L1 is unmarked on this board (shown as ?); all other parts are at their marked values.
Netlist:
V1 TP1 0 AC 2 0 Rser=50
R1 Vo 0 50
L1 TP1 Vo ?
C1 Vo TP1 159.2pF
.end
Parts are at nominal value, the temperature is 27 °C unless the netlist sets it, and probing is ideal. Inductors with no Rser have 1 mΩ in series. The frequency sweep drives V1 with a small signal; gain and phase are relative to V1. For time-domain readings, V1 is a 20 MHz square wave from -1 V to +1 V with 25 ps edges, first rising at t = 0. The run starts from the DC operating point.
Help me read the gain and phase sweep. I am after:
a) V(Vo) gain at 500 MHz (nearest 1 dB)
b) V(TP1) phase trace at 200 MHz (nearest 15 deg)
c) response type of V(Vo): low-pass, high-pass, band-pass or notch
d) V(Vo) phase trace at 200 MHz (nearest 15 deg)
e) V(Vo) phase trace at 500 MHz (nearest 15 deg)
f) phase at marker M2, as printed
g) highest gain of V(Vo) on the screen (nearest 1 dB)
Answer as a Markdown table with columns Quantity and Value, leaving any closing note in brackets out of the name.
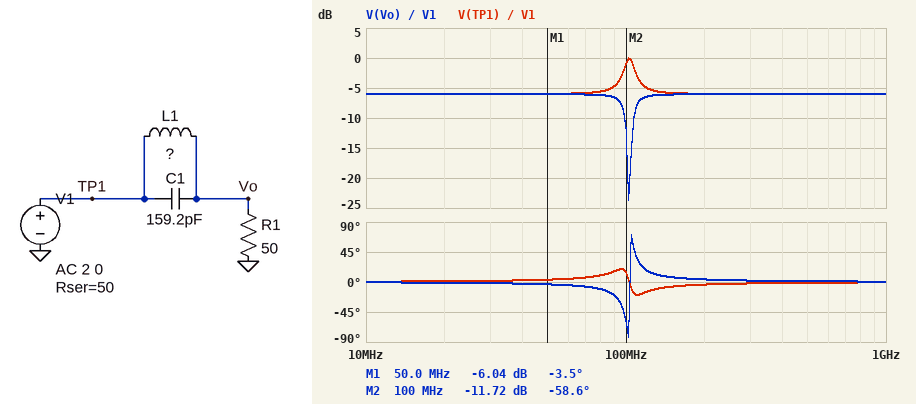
| Quantity | Value |
|---|---|
| V(Vo) gain at 500 MHz | -6 dB |
| V(TP1) phase trace at 200 MHz | 0 deg |
| response type of V(Vo): low-pass, high-pass, band-pass or notch | notch |
| V(Vo) phase trace at 200 MHz | 0 deg |
| V(Vo) phase trace at 500 MHz | 0 deg |
| phase at marker M2, as printed | -58.6 deg |
| highest gain of V(Vo) on the screen | -6 dB |
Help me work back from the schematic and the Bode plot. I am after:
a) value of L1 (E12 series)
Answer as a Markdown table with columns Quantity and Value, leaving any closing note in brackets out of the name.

| Quantity | Value |
|---|---|
| value of L1 | 15 nH |
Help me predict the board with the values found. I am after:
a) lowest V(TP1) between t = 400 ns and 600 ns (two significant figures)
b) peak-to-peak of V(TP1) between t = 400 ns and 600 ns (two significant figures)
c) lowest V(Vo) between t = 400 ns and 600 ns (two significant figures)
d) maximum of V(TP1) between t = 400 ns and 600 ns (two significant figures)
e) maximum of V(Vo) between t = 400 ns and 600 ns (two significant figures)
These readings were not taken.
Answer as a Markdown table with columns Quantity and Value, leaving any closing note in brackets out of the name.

| Quantity | Value |
|---|---|
| lowest V(TP1) between t = 400 ns and 600 ns | -650 mV |
| peak-to-peak of V(TP1) between t = 400 ns and 600 ns | 1.3 V |
| lowest V(Vo) between t = 400 ns and 600 ns | -630 mV |
| maximum of V(TP1) between t = 400 ns and 600 ns | 650 mV |
| maximum of V(Vo) between t = 400 ns and 600 ns | 630 mV |
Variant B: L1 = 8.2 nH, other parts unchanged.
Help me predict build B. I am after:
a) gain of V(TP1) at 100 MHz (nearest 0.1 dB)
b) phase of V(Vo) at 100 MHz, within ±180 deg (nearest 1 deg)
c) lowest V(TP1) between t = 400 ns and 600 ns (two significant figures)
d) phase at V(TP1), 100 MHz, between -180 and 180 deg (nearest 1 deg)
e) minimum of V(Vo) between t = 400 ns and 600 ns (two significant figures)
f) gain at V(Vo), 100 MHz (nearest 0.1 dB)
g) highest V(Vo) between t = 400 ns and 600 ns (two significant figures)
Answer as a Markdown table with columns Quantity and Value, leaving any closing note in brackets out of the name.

| Quantity | Value |
|---|---|
| gain of V(TP1) at 100 MHz | -5.9 dB |
| phase of V(Vo) at 100 MHz, within ±180 deg | -6 deg |
| lowest V(TP1) between t = 400 ns and 600 ns | -620 mV |
| phase at V(TP1), 100 MHz, between -180 and 180 deg | 6 deg |
| minimum of V(Vo) between t = 400 ns and 600 ns | -610 mV |
| gain at V(Vo), 100 MHz | -6.1 dB |
| highest V(Vo) between t = 400 ns and 600 ns | 610 mV |
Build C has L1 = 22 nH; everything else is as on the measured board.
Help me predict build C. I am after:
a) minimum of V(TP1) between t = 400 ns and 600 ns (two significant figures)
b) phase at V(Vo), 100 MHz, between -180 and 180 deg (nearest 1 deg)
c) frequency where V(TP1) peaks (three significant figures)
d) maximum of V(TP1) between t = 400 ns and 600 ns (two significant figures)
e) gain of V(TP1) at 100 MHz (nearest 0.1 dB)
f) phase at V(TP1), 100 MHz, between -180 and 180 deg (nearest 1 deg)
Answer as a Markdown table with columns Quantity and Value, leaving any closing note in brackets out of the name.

| Quantity | Value |
|---|---|
| minimum of V(TP1) between t = 400 ns and 600 ns | -580 mV |
| phase at V(Vo), 100 MHz, between -180 and 180 deg | 20 deg |
| frequency where V(TP1) peaks | 85.0 MHz |
| maximum of V(TP1) between t = 400 ns and 600 ns | 580 mV |
| gain of V(TP1) at 100 MHz | -4.7 dB |
| phase at V(TP1), 100 MHz, between -180 and 180 deg | -16 deg |
